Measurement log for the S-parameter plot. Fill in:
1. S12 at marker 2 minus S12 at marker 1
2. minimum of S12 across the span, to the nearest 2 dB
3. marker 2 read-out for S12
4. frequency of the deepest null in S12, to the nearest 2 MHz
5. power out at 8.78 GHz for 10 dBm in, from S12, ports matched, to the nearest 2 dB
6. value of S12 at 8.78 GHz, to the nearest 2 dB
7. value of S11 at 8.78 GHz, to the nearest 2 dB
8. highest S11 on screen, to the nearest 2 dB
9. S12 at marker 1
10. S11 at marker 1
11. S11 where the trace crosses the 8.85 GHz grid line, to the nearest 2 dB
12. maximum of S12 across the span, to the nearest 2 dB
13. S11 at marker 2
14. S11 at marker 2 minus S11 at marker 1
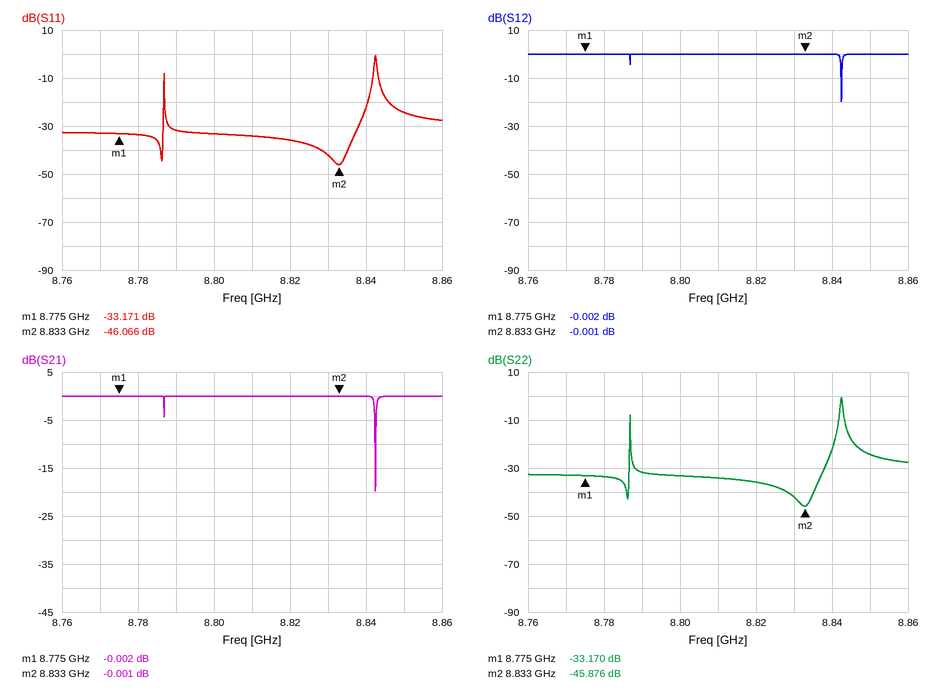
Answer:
0.001 dB
-20 dB
-0.001 dB
8.842 GHz
10 dBm
0 dB
-34 dB
0 dB
-0.002 dB
-33.171 dB
-24 dB
0 dB
-46.066 dB
-12.895 dB
